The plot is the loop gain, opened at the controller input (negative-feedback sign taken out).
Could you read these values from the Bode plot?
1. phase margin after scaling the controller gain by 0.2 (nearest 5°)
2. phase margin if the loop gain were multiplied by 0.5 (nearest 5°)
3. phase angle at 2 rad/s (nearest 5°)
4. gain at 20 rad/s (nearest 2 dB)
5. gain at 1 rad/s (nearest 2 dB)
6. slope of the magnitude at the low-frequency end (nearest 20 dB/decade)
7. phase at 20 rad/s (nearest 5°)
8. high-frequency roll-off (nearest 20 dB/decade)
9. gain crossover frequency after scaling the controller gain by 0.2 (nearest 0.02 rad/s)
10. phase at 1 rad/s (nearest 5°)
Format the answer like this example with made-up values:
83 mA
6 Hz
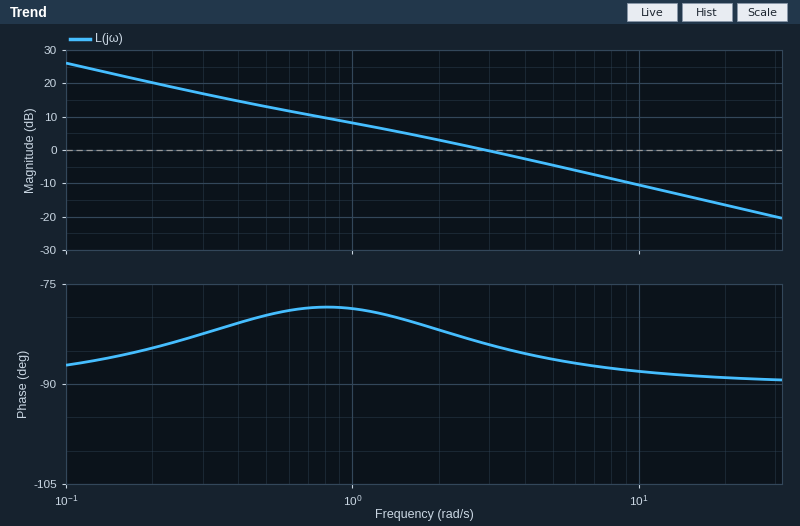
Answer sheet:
100°
100°
-80°
-16 dB
8 dB
-20 dB/decade
-90°
-20 dB/decade
0.44 rad/s
-80°
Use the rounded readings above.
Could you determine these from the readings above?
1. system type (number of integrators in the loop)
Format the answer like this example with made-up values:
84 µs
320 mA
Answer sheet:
1
